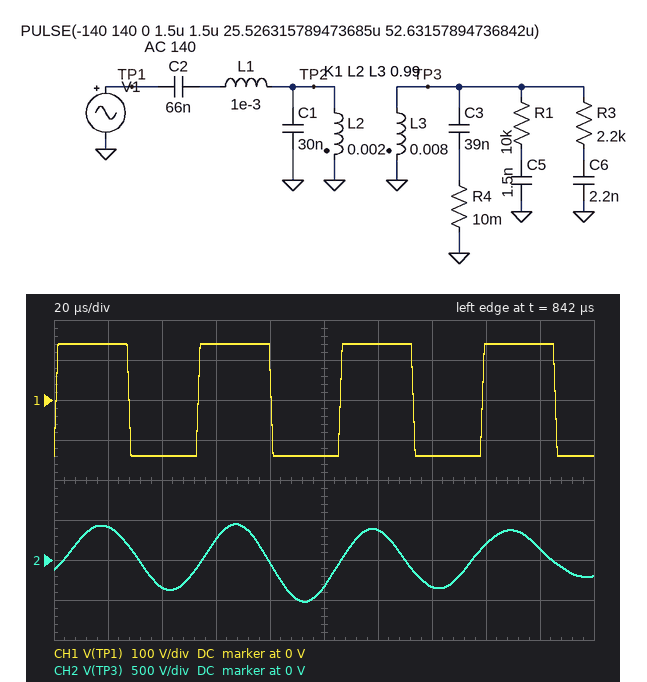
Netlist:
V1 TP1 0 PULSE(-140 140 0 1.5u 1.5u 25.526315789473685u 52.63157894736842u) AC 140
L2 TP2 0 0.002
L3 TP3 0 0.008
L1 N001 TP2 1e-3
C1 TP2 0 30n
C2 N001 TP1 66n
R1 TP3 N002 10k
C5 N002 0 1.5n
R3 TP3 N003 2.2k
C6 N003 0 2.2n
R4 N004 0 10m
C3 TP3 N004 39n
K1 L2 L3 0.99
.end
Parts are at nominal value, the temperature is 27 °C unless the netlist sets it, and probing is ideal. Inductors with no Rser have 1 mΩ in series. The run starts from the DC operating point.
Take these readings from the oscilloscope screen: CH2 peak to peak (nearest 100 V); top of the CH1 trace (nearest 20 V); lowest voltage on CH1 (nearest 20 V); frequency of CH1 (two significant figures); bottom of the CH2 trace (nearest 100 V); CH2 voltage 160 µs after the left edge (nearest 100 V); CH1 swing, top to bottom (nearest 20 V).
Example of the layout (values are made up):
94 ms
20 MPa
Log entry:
1.0 kV
140 V
-140 V
19 kHz
-500 V
200 V
280 V
